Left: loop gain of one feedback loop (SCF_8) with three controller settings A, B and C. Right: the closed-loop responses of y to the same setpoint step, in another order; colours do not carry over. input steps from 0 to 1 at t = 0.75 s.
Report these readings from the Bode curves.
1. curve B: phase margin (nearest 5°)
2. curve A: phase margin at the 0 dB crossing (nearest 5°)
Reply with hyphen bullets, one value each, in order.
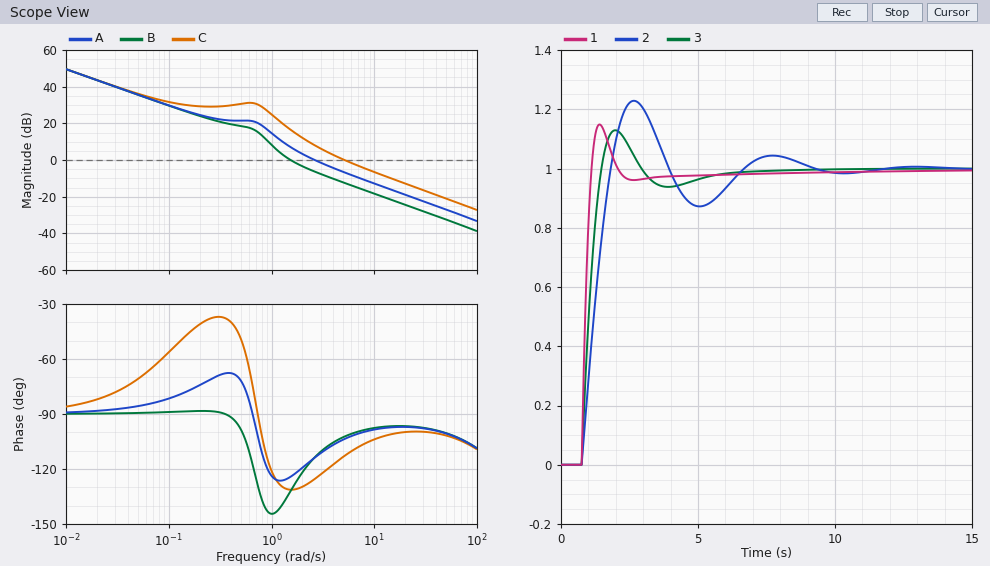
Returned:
- 50°
- 65°
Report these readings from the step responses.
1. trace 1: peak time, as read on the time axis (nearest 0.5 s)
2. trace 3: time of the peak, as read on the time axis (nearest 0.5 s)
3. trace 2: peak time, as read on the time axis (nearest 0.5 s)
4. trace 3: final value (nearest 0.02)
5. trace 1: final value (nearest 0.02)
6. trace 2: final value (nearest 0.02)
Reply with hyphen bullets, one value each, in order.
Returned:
- 1.5 s
- 2.0 s
- 2.5 s
- 1.00
- 1.00
- 1.00
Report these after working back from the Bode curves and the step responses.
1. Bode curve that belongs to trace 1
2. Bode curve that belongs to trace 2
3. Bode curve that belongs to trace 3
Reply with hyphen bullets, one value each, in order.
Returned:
- C
- B
- A
